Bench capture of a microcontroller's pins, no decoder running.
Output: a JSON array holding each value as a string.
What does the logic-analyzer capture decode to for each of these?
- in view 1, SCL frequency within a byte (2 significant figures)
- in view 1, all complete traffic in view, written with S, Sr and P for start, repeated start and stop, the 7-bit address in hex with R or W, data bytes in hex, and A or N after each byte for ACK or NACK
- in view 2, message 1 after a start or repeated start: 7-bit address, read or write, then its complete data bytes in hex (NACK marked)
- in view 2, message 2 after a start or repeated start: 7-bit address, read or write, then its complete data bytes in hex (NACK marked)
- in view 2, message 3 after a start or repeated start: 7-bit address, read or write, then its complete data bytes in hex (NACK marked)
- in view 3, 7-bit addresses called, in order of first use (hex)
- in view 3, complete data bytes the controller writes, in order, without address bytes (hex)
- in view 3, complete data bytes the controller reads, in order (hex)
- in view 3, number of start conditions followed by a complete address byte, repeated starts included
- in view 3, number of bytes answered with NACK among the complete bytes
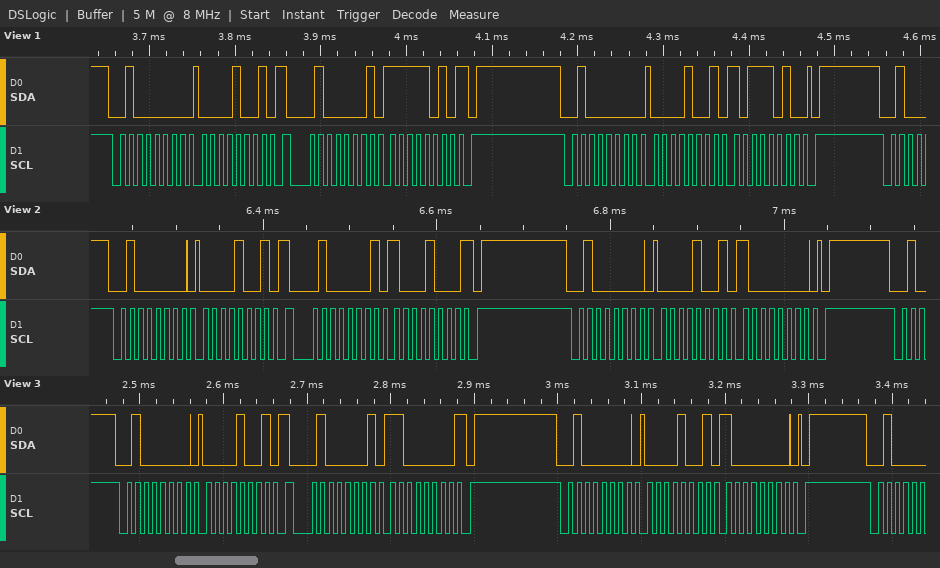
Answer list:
["100 kHz", "S 20W A 09 A Sr 20R A FA N P S 20W A 09 A BA A P", "0x20 write: 09", "0x20 read: 88 NACK", "0x20 write: 09 80", "0x20", "09 09 80", "C0", "3", "1"]
